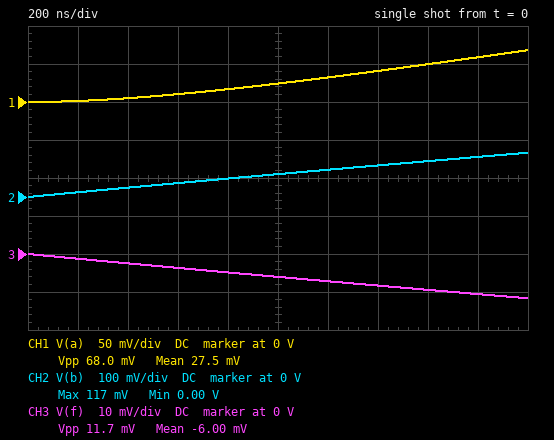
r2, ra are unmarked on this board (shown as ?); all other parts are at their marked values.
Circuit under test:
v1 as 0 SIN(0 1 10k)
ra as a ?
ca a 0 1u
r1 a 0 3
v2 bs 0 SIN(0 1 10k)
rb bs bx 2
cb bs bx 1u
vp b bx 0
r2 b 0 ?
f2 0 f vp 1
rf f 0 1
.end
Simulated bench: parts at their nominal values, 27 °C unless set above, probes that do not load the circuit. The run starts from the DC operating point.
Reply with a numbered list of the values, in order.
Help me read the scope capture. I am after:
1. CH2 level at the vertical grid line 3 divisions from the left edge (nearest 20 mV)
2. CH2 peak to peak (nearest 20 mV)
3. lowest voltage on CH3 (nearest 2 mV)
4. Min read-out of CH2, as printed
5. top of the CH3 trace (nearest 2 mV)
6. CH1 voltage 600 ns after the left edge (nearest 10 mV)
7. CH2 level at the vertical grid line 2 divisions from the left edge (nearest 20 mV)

1. 40 mV
2. 120 mV
3. -12 mV
4. 0.00 V
5. 0 V
6. 10 mV
7. 20 mV
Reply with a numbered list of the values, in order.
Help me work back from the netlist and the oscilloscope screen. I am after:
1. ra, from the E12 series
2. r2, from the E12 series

1. 0.82 Ω
2. 10 Ω
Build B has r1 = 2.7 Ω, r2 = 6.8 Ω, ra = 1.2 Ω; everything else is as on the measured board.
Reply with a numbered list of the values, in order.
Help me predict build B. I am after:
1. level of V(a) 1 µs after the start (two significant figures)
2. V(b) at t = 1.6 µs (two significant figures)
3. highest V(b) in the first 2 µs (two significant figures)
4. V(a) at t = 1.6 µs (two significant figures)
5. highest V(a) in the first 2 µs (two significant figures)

1. 18 mV
2. 92 mV
3. 110 mV
4. 39 mV
5. 54 mV
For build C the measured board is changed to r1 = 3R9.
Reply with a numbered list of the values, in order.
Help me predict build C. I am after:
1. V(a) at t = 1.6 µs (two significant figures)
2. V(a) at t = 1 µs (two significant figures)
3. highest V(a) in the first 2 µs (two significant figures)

1. 51 mV
2. 25 mV
3. 70 mV
